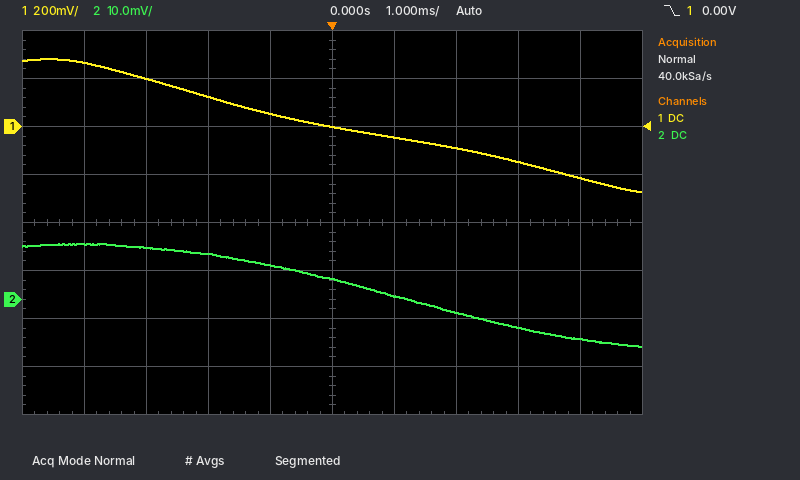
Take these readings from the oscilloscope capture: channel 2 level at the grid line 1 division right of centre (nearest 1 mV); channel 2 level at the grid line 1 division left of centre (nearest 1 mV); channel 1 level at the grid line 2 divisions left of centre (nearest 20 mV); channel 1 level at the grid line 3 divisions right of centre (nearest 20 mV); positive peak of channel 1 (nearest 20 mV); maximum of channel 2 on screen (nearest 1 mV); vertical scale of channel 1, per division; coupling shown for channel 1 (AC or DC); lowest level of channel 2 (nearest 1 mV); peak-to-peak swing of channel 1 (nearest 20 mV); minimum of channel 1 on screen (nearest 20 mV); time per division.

1 mV
7 mV
120 mV
-140 mV
280 mV
12 mV
200 mV
DC
-10 mV
560 mV
-280 mV
1 ms
